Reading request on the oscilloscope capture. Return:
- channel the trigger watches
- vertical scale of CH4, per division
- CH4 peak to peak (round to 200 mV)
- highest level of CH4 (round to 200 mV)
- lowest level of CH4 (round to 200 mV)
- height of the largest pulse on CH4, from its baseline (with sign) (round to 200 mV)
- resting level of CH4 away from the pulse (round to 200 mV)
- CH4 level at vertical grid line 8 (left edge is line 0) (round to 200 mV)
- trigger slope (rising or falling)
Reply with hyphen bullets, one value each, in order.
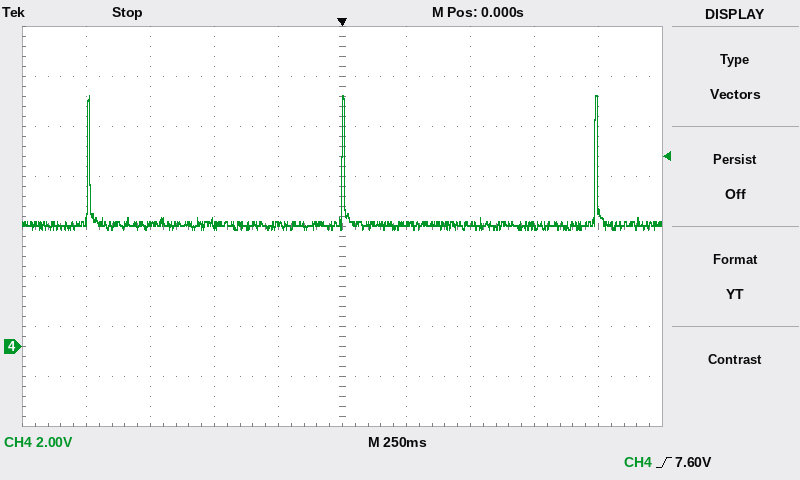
- CH4
- 2 V
- 5.4 V
- 10.0 V
- 4.6 V
- +5.2 V
- 4.8 V
- 4.8 V
- rising
